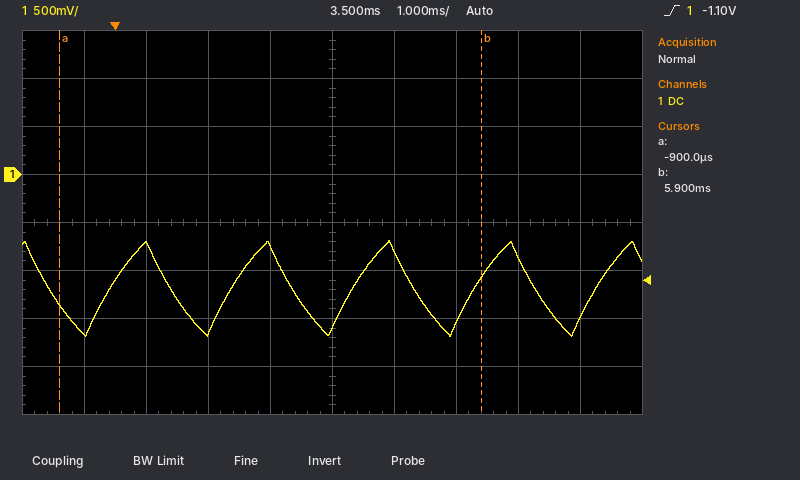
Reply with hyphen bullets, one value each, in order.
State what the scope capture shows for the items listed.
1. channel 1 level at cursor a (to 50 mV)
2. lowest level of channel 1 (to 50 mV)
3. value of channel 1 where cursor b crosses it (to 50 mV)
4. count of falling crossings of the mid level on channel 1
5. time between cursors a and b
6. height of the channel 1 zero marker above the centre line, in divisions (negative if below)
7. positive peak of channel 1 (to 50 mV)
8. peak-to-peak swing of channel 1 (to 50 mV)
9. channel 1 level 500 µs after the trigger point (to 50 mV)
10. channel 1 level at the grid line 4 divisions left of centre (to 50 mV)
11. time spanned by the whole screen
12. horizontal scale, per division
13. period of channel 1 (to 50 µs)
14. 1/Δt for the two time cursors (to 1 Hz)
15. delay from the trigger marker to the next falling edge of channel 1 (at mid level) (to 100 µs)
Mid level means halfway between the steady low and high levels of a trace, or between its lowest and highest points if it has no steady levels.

- -1.35 V
- -1.70 V
- -1.05 V
- 5
- 6.8 ms
- +1.0 div
- -700 mV
- 1.00 V
- -750 mV
- -1.65 V
- 10 ms
- 1 ms
- 1.95 ms
- 147 Hz
- 900 µs
